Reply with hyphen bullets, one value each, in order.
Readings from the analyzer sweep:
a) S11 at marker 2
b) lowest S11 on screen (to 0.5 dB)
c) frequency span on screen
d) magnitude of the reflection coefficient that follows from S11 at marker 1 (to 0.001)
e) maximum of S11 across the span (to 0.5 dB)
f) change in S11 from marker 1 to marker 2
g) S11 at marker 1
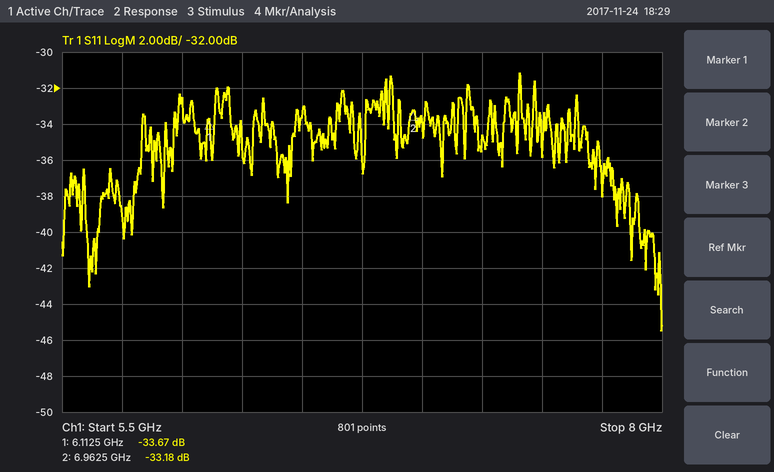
- -33.18 dB
- -45.5 dB
- 2.5 GHz
- 0.021
- -31.0 dB
- 0.49 dB
- -33.67 dB
